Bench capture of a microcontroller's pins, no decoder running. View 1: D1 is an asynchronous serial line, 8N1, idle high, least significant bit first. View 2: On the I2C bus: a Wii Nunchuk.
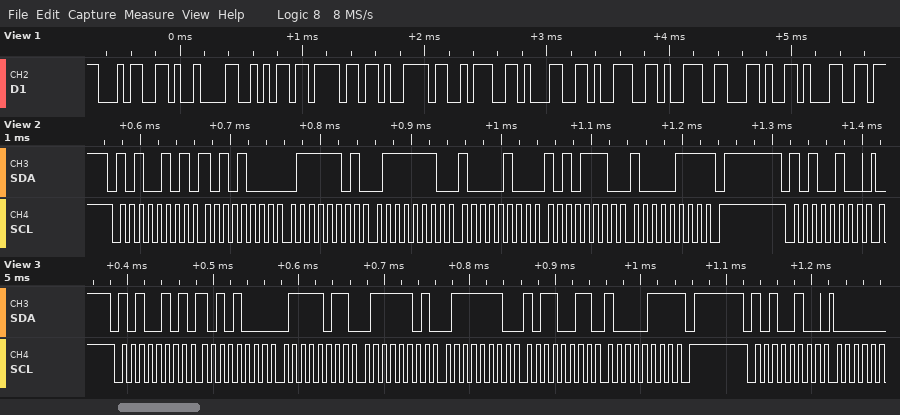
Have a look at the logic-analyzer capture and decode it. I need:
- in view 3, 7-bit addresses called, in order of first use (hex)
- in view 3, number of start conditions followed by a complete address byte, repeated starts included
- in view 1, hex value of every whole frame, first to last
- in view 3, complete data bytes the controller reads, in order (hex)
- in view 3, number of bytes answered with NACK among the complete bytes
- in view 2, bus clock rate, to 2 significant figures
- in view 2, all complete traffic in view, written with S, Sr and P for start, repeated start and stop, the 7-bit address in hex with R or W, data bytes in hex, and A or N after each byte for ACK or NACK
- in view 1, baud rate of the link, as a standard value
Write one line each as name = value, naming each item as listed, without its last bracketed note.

in view 3, 7-bit addresses called, in order of first use = 0x52
in view 3, number of start conditions followed by a complete address byte, repeated starts included = 2
in view 1, hex value of every whole frame, first to last = 0x34 0x09 0x6A 0x6F 0x79 0x3A 0x31 0x39 0x39 0x2C 0x31
in view 3, complete data bytes the controller reads, in order = A8 7B 7D 7E B3 87
in view 3, number of bytes answered with NACK among the complete bytes = 1
in view 2, bus clock rate, to 2 significant figures = 100 kHz
in view 2, all complete traffic in view, written with S, Sr and P for start, repeated start and stop, the 7-bit address in hex with R or W, data bytes in hex, and A or N after each byte for ACK or NACK = S 52R A A8 A 7D A 7E A 84 A AE A 87 N P S 52W A
in view 1, baud rate of the link, as a standard value = 19200 baud
